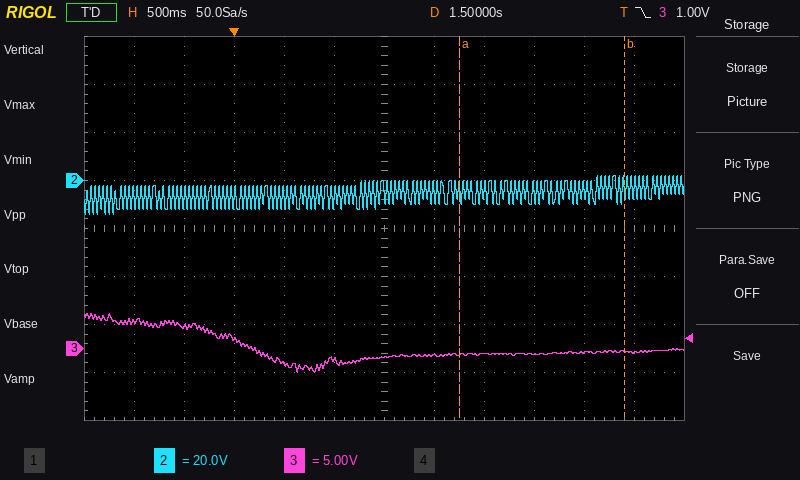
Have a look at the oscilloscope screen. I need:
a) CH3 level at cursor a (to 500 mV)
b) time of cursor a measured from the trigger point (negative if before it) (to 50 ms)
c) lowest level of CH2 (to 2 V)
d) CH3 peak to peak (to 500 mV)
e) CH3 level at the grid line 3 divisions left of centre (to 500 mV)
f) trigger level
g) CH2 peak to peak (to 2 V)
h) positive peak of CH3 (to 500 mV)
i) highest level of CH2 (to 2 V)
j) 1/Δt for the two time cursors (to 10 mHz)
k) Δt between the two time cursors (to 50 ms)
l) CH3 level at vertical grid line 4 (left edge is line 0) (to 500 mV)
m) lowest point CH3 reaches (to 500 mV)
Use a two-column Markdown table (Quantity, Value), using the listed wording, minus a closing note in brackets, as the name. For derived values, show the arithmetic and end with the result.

| Quantity | Value |
|---|---|
| CH3 level at cursor a | -500 mV |
| time of cursor a measured from the trigger point (negative if before it) | +2.25 s |
| lowest level of CH2 | -14 V |
| CH3 peak to peak | 3.5 V − (-2.5 V) = 6.0 V |
| CH3 level at the grid line 3 divisions left of centre | 1.0 V |
| trigger level | 1.00 V |
| CH2 peak to peak | 2 V − (-14 V) = 16 V |
| positive peak of CH3 | 3.5 V |
| highest level of CH2 | 2 V |
| 1/Δt for the two time cursors | 1 / 1.65 s ≈ 610 mHz |
| Δt between the two time cursors | 1.65 s |
| CH3 level at vertical grid line 4 (left edge is line 0) | -1.5 V |
| lowest point CH3 reaches | -2.5 V |
